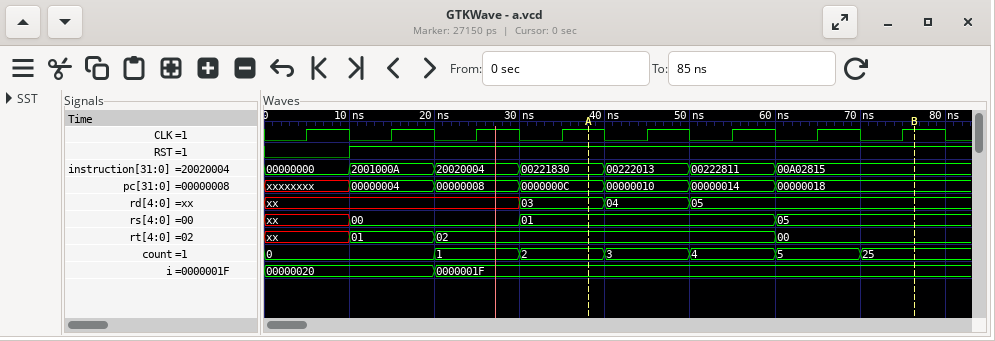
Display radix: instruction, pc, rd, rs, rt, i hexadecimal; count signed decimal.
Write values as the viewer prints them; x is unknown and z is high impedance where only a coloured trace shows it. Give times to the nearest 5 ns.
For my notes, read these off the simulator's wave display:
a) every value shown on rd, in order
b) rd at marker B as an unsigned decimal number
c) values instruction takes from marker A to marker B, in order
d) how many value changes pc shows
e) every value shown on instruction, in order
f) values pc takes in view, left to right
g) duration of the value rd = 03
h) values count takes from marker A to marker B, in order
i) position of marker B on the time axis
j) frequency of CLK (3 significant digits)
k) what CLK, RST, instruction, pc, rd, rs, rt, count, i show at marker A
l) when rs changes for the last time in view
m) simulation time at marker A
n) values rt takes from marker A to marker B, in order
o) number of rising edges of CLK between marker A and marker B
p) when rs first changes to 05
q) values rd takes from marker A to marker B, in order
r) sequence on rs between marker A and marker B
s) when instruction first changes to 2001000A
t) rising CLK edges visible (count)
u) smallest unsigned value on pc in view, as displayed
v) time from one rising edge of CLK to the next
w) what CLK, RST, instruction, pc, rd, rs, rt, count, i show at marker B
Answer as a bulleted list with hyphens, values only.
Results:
- xx, 03, 04, 05
- 5
- 00221830, 00222013, 00222811, 00A02815
- 6
- 00000000, 2001000A, 20020004, 00221830, 00222013, 00222811, 00A02815
- xxxxxxxx, 00000004, 00000008, 0000000C, 00000010, 00000014, 00000018
- 10 ns
- 2, 3, 4, 5, 25
- 75 ns
- 100 MHz
- CLK=1, RST=1, instruction=00221830, pc=0000000C, rd=03, rs=01, rt=02, count=2, i=0000001F
- 60 ns
- 40 ns
- 02, 00
- 4
- 60 ns
- 03, 04, 05
- 01, 05
- 10 ns
- 8
- 00000004
- 10 ns
- CLK=1, RST=1, instruction=00A02815, pc=00000018, rd=05, rs=05, rt=00, count=25, i=0000001F
